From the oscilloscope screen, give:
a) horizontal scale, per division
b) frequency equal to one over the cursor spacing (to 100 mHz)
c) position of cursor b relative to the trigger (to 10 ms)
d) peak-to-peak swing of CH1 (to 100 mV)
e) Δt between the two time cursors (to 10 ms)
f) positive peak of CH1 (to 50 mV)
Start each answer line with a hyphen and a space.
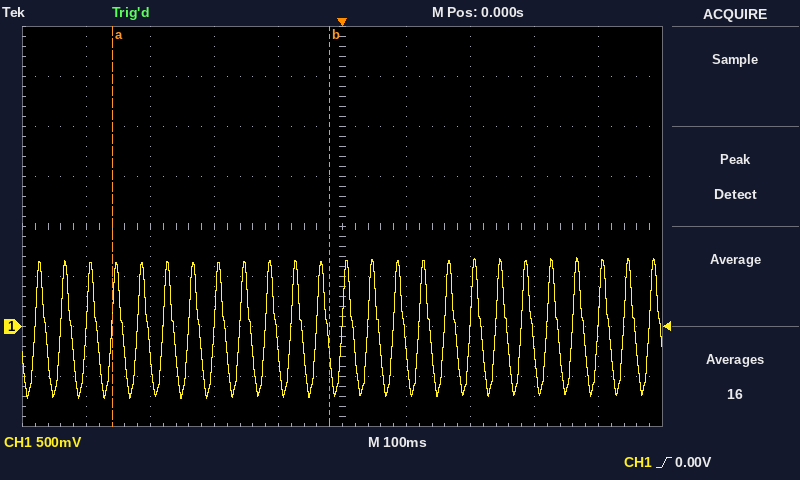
- 100 ms
- 2.9 Hz
- -20 ms
- 1.40 V
- 340 ms
- 700 mV
